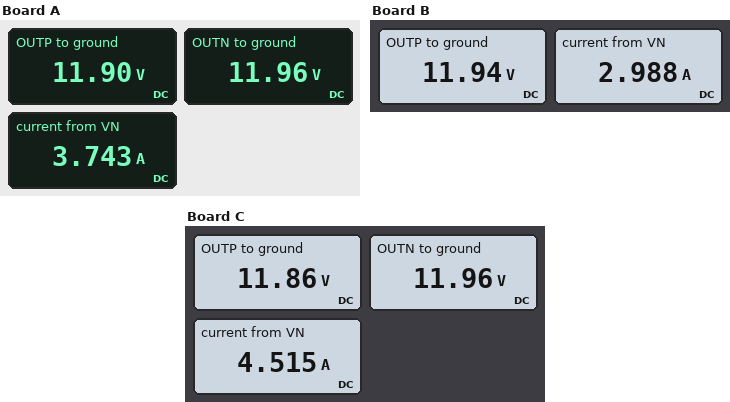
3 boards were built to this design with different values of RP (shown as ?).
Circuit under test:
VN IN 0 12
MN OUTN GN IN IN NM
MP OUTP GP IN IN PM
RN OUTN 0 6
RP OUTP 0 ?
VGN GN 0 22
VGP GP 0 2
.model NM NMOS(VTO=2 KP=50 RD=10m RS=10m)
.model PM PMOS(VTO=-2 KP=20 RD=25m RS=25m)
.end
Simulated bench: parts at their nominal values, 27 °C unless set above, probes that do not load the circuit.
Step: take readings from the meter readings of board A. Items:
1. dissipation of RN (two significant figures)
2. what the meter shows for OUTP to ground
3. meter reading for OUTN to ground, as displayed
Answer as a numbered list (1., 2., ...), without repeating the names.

1. 24 W
2. 11.90 V
3. 11.96 V
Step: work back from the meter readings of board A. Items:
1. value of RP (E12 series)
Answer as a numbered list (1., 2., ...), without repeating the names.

1. 6.8 Ω
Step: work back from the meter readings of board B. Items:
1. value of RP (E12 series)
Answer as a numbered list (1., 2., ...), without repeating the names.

1. 12 Ω
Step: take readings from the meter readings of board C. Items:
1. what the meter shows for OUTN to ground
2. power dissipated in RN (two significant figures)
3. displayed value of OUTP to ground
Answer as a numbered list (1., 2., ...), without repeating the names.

1. 11.96 V
2. 24 W
3. 11.86 V
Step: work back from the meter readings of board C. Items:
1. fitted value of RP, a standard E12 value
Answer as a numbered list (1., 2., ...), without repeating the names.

1. 4.7 Ω
